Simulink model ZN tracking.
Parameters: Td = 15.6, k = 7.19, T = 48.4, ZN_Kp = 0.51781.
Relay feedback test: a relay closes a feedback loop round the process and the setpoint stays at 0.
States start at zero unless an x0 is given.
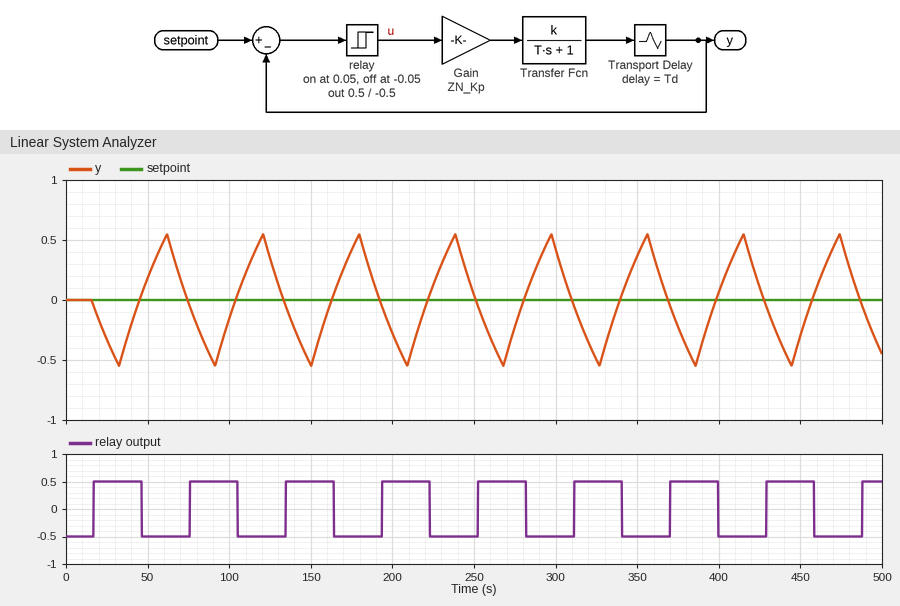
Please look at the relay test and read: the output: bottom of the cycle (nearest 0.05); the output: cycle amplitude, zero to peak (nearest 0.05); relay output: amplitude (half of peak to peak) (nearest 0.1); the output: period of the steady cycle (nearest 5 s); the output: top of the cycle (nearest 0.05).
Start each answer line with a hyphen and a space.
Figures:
- -0.55
- 0.55
- 0.5
- 60 s
- 0.55
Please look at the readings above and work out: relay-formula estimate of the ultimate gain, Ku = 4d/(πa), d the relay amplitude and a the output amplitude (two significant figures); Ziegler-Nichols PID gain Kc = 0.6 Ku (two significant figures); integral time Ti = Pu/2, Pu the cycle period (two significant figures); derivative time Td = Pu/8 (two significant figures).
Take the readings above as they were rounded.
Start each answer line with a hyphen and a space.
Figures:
- 1.2
- 0.72
- 30 s
- 7.5 s
